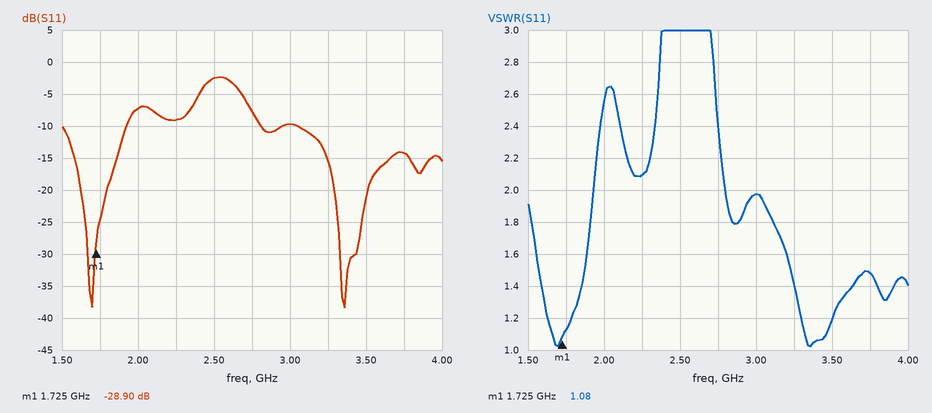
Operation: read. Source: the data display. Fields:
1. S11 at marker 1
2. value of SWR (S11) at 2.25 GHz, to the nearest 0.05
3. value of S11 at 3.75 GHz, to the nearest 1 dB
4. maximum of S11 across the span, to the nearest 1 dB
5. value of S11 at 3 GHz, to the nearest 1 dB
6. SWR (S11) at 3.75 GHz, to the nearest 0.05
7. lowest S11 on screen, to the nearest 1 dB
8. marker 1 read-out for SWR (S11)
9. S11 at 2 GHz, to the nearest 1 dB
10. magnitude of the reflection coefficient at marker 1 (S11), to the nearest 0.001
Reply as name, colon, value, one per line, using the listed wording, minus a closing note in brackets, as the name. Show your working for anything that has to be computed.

S11 at marker 1: -28.90 dB
value of SWR (S11) at 2.25 GHz, to the nearest 0.05: 2.10
value of S11 at 3.75 GHz, to the nearest 1 dB: -14 dB
maximum of S11 across the span, to the nearest 1 dB: -2 dB
value of S11 at 3 GHz, to the nearest 1 dB: -10 dB
SWR (S11) at 3.75 GHz, to the nearest 0.05: 1.50
lowest S11 on screen, to the nearest 1 dB: -38 dB
marker 1 read-out for SWR: 1.08
S11 at 2 GHz, to the nearest 1 dB: -7 dB
magnitude of the reflection coefficient at marker 1 (S11), to the nearest 0.001: 10^(-28.9/20) ≈ 0.036
